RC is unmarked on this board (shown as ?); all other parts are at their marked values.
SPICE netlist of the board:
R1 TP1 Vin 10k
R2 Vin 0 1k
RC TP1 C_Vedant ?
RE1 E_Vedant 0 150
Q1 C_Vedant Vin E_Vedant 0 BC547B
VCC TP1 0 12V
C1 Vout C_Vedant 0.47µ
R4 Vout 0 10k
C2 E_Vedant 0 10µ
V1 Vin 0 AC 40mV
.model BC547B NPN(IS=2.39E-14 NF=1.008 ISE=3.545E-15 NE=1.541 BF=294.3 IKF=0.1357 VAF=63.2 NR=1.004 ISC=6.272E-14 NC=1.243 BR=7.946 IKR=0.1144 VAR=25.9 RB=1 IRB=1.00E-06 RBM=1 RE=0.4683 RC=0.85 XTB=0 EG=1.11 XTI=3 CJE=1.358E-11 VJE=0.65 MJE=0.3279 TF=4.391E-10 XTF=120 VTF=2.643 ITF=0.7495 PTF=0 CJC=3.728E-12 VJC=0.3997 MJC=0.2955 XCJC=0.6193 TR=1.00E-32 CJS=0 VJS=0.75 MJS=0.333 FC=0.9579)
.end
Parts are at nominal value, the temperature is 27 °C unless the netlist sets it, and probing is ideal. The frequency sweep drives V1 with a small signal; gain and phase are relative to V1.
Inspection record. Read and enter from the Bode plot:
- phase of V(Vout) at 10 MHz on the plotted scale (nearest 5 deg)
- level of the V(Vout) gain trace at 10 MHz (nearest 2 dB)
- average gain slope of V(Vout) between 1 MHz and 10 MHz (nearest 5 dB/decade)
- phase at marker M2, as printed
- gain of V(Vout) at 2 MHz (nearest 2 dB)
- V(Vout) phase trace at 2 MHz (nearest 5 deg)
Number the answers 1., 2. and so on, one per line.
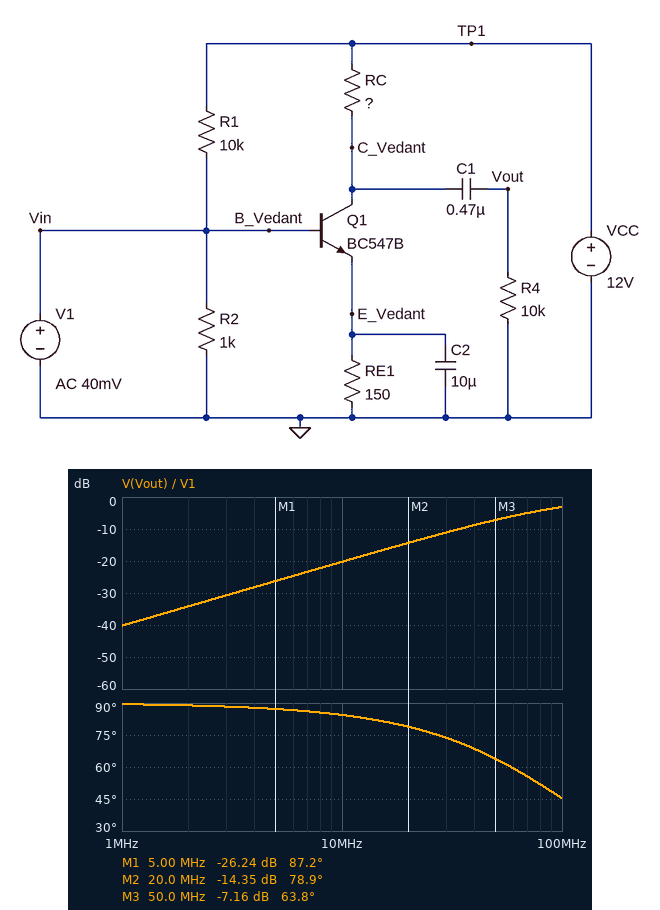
1. 85 deg
2. -20 dB
3. 20 dB/decade
4. 78.9 deg
5. -34 dB
6. 90 deg
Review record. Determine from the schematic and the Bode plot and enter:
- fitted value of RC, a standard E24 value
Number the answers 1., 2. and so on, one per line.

1. 1.3 kΩ
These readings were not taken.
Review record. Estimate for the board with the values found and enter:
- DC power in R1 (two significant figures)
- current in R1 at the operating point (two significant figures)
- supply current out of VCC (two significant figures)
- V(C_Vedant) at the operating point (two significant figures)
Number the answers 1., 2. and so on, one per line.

1. 14 mW
2. 1.2 mA
3. 1.2 mA
4. 12 V
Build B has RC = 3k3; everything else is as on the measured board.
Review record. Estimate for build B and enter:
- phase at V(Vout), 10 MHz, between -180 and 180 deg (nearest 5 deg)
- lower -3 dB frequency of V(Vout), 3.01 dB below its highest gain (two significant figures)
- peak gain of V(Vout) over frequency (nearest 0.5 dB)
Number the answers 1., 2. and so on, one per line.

1. 80 deg
2. 47 MHz
3. 0 dB
